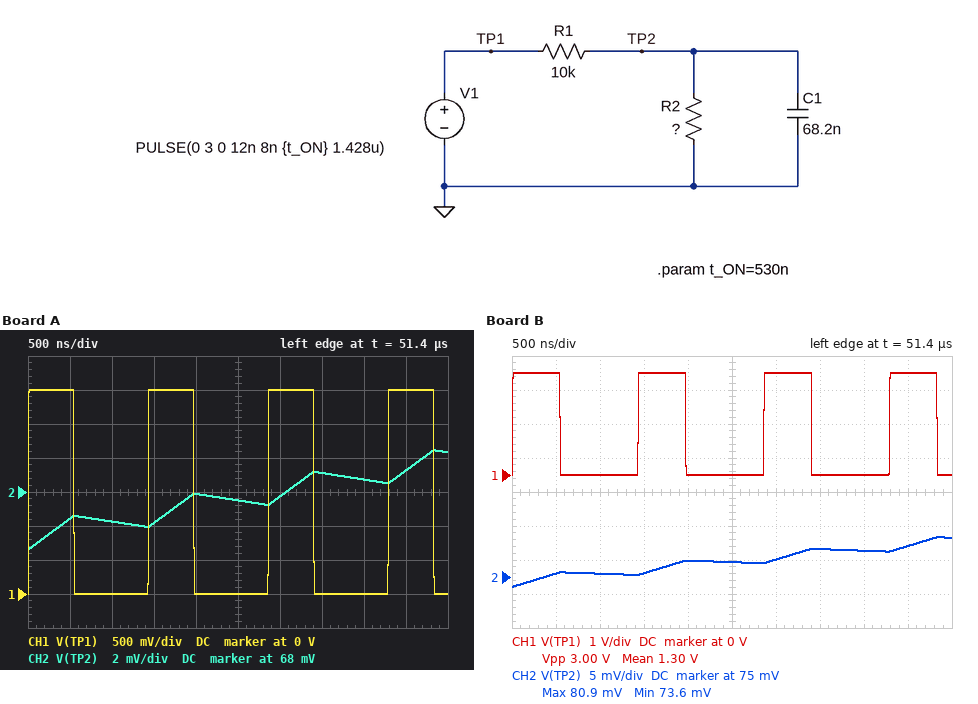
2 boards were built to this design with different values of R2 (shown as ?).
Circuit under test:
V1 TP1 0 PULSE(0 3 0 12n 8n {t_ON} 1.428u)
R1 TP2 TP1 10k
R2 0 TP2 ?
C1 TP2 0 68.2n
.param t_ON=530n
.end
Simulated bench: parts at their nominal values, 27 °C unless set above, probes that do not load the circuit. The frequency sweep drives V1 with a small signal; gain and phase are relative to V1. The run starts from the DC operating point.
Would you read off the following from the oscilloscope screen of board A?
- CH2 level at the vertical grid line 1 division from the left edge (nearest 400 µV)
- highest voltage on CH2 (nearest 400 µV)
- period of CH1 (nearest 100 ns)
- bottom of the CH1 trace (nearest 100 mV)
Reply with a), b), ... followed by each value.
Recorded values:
a) 66.4 mV
b) 70.4 mV
c) 1.4 µs
d) 0 V
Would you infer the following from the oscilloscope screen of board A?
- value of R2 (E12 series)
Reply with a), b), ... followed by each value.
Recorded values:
a) 1.5 kΩ
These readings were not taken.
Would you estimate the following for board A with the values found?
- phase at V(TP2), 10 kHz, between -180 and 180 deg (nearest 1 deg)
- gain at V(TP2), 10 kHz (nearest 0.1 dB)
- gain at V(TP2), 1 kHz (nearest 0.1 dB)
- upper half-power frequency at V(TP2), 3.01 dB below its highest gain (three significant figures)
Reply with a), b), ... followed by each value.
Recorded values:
a) -80 deg
b) -32.8 dB
c) -18.9 dB
d) 1.79 kHz
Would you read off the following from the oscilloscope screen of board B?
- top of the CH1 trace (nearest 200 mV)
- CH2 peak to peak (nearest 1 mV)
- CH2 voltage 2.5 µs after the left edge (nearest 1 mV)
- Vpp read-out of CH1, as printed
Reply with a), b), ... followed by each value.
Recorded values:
a) 3.0 V
b) 7 mV
c) 77 mV
d) 3.00 V
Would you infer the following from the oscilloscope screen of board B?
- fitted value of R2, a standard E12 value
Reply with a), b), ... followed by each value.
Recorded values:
a) 3.3 kΩ
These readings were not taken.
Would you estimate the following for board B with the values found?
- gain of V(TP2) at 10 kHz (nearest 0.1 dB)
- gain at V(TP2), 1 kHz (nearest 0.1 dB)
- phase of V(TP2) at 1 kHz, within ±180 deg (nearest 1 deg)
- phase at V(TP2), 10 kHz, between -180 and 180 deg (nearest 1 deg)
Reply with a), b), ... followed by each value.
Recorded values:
a) -32.7 dB
b) -15.4 dB
c) -47 deg
d) -85 deg
